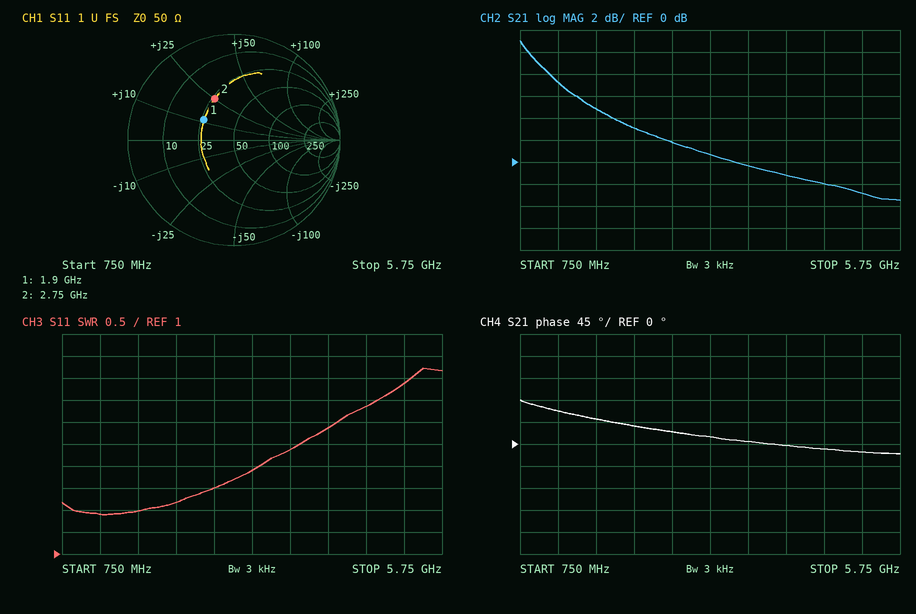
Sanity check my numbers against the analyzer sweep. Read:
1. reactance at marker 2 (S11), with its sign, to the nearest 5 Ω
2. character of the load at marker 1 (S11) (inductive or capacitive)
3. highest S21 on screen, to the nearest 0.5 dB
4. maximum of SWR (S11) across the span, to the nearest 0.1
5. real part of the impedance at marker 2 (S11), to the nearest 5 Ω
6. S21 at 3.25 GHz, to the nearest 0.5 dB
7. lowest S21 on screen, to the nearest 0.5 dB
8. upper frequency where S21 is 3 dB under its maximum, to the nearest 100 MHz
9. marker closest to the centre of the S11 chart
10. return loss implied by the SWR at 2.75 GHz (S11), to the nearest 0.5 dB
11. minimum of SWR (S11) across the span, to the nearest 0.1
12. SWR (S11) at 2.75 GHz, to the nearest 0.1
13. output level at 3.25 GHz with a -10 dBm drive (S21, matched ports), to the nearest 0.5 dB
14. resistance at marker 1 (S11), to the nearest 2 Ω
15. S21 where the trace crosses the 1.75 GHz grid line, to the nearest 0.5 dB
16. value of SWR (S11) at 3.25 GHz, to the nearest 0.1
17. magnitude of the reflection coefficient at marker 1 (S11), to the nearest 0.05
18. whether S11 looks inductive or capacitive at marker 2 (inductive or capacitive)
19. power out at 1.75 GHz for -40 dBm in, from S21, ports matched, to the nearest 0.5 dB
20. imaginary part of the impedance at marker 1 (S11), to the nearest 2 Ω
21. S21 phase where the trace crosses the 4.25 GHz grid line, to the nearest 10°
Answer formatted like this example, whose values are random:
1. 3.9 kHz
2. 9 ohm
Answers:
1. +25 Ω
2. inductive
3. 11.0 dB
4. 5.2
5. 25 Ω
6. 0.5 dB
7. -3.5 dB
8. 1.1 GHz
9. marker 1
10. 7.5 dB
11. 1.9
12. 2.5
13. -9.5 dBm
14. 26 Ω
15. 5.0 dB
16. 2.9
17. 0.35
18. inductive
19. -35.0 dBm
20. +12 Ω
21. 0°
